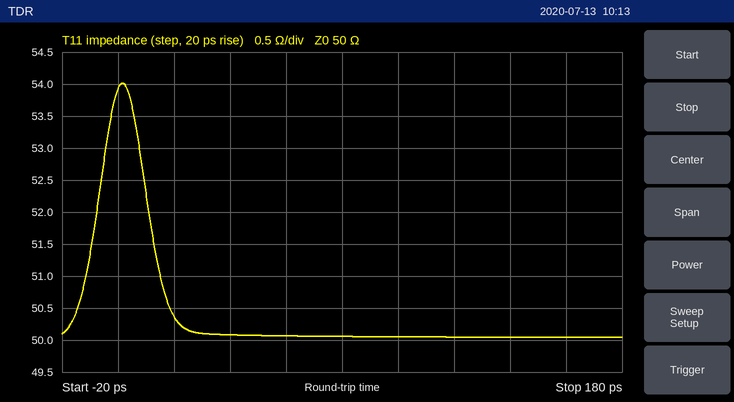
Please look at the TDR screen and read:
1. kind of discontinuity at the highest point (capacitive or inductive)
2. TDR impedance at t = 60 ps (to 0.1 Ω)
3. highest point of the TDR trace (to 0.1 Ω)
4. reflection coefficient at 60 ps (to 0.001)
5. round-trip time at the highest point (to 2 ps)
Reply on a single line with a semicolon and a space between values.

inductive; 50.1 Ω; 54.0 Ω; +0.001; 2 ps
